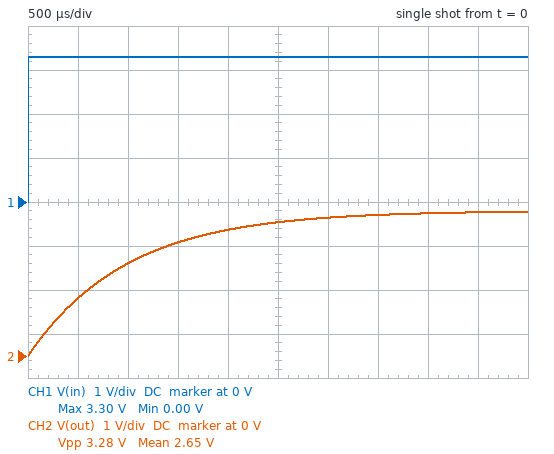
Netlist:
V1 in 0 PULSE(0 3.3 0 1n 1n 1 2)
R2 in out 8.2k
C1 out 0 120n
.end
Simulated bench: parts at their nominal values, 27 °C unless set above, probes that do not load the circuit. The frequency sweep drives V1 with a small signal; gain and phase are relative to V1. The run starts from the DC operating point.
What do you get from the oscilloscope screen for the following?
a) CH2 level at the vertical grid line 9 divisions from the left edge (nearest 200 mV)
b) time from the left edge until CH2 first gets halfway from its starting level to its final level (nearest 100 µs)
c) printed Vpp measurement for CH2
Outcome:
3.2 V
700 µs
3.28 V
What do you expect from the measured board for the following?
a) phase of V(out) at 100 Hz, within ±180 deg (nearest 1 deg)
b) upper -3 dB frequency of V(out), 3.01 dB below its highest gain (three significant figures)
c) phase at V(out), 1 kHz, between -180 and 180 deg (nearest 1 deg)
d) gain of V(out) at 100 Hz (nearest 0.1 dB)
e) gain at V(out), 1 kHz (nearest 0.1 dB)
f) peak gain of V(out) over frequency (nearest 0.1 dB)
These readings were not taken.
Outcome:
-32 deg
162 Hz
-81 deg
-1.4 dB
-15.9 dB
0 dB
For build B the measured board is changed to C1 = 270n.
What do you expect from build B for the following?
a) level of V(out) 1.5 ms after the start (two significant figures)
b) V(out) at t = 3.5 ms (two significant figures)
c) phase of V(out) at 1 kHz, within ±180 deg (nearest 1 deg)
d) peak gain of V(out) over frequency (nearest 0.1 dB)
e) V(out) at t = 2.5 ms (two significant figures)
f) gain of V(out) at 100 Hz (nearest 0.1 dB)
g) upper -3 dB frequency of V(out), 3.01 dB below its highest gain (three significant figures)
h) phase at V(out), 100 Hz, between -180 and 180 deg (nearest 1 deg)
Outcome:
1.6 V
2.6 V
-86 deg
0 dB
2.2 V
-4.7 dB
71.9 Hz
-54 deg
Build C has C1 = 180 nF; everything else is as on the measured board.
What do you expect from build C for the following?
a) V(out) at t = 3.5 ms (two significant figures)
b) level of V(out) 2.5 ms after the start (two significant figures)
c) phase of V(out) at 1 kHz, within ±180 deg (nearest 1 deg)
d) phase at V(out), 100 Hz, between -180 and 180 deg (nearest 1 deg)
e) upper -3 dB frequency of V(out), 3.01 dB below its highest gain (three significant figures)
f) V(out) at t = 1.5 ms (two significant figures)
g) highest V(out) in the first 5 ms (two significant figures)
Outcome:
3.0 V
2.7 V
-84 deg
-43 deg
108 Hz
2.1 V
3.2 V
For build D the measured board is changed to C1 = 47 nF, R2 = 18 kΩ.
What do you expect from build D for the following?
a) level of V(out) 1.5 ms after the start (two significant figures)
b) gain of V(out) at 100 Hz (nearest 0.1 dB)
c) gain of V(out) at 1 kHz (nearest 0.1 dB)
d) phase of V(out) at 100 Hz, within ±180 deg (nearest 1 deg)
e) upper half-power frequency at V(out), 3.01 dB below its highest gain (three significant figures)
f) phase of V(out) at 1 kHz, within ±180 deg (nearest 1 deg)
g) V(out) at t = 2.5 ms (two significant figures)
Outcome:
2.7 V
-1.1 dB
-14.7 dB
-28 deg
188 Hz
-79 deg
3.1 V
